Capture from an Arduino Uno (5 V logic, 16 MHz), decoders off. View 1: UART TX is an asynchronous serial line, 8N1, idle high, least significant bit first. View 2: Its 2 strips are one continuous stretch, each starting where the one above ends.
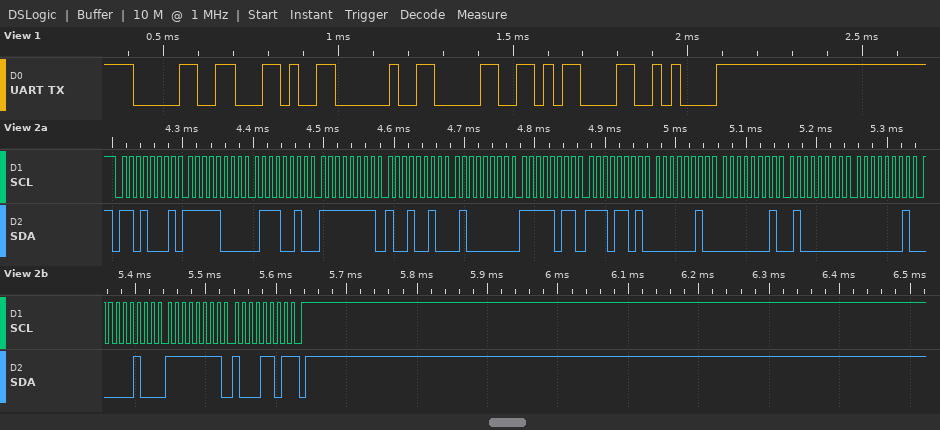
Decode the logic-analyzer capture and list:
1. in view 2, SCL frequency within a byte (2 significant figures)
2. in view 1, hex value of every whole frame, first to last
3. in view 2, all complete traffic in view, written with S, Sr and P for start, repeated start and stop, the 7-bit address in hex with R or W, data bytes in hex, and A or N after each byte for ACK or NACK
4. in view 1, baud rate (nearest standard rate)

100 kHz
30 2C 20 30 0D 0A
S 68R A F8 A 72 A FF A 92 A 40 A FB A ED A 02 A 01 A 40 A 01 A 04 A FF A 8D N P
38400 baud
